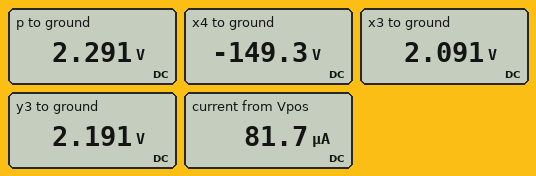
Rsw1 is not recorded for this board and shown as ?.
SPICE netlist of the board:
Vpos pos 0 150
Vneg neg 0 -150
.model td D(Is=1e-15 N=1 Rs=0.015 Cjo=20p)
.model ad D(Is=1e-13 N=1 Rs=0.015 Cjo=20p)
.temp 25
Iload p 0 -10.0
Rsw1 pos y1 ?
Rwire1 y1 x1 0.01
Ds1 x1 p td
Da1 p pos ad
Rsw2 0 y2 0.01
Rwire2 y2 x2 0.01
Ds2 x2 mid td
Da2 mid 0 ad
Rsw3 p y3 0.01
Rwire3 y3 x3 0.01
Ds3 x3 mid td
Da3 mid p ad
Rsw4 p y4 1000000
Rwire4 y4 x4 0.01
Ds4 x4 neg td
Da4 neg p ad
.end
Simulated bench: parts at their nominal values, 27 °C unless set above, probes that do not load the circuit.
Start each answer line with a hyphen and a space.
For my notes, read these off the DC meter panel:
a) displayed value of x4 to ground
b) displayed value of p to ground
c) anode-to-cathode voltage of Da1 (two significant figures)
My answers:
- -149.3 V
- 2.291 V
- -150 V
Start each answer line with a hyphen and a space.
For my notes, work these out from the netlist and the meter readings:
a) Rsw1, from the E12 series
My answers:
- 1.8 MΩ
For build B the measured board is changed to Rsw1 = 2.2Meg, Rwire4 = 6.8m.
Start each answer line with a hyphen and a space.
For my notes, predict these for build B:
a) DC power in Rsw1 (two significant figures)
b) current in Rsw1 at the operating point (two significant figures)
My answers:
- 9.8 mW
- 67 µA
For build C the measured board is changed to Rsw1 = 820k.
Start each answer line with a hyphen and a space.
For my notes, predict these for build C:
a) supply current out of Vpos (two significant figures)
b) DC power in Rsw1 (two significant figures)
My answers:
- 180 µA
- 26 mW
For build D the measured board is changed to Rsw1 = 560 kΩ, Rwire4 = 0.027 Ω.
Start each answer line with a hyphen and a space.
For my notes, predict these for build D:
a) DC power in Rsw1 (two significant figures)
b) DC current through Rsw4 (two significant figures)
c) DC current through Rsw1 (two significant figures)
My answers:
- 39 mW
- 150 µA
- 260 µA
